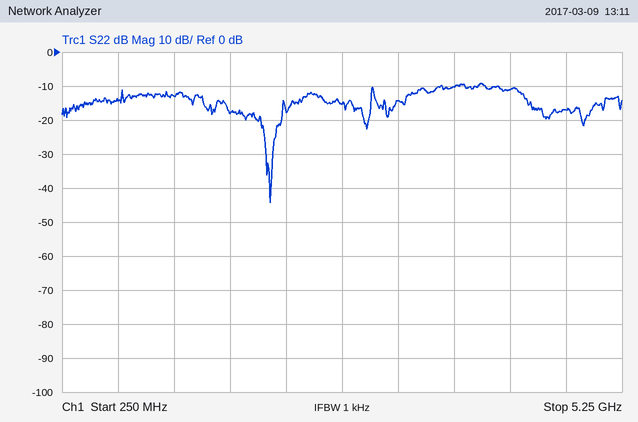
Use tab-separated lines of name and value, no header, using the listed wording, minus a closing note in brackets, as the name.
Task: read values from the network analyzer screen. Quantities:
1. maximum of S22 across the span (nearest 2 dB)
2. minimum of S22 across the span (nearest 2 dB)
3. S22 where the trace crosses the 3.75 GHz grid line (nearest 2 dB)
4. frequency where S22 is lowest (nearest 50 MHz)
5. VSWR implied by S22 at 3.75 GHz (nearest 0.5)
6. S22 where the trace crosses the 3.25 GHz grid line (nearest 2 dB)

maximum of S22 across the span	-10 dB
minimum of S22 across the span	-44 dB
S22 where the trace crosses the 3.75 GHz grid line	-10 dB
frequency where S22 is lowest	2.10 GHz
VSWR implied by S22 at 3.75 GHz	2.0
S22 where the trace crosses the 3.25 GHz grid line	-14 dB
